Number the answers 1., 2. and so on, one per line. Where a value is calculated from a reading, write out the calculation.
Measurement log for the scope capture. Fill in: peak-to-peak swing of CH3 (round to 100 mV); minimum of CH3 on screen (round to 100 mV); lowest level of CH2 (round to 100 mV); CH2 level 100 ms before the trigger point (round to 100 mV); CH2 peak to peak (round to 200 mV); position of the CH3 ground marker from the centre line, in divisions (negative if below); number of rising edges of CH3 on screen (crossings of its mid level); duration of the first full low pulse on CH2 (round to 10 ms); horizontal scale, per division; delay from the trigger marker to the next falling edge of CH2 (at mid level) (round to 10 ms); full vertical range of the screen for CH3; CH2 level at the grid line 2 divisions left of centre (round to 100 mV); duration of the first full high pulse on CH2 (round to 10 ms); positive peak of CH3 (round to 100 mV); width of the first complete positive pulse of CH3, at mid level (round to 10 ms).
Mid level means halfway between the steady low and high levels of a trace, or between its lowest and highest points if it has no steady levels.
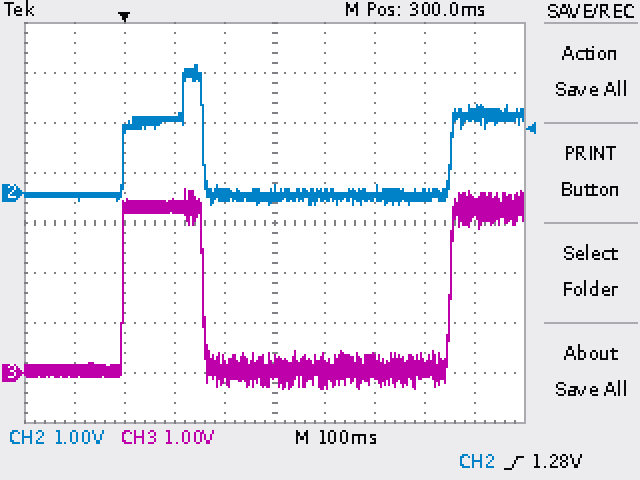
1. 3.7 V − (-300 mV) = 4.0 V
2. -300 mV
3. -200 mV
4. 0.0 V
5. 2.8 V
6. -3.0 div
7. 2
8. 490 ms
9. 100 ms
10. 160 ms
11. 8 V
12. 1.5 V
13. 160 ms
14. 3.7 V
15. 160 ms
